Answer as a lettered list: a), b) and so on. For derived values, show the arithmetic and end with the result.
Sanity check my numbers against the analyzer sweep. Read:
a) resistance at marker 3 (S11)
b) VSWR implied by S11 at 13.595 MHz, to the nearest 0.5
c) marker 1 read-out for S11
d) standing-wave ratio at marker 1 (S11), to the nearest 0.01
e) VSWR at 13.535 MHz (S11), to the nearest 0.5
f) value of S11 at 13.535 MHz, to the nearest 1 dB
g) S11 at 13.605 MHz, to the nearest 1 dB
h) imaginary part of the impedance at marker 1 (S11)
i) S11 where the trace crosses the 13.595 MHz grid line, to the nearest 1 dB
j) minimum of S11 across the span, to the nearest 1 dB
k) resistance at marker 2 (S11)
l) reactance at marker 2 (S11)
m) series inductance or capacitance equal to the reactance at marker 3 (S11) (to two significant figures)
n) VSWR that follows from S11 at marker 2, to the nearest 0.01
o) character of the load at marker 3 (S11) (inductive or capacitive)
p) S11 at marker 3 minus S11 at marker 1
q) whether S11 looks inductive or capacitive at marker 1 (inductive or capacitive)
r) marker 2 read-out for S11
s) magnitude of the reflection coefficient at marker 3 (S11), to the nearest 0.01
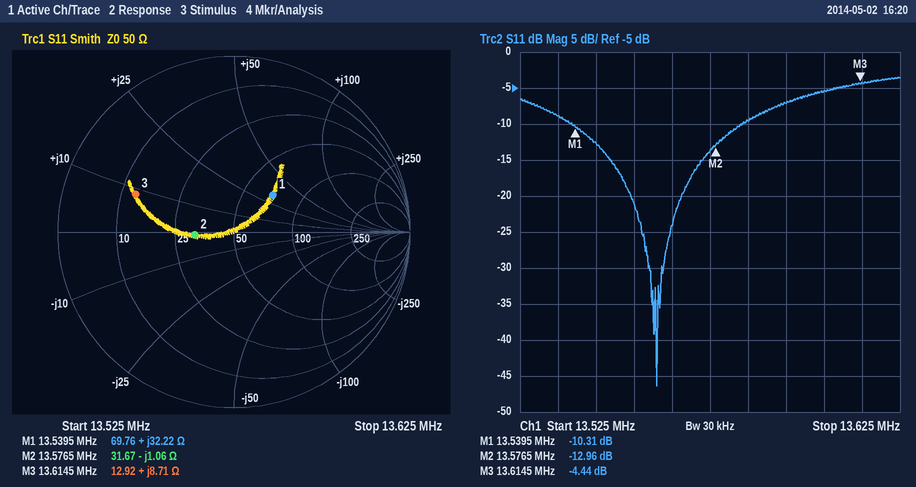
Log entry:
a) 12.92 Ω
b) |Γ| = 10^(-7/20) = 0.4467; VSWR = (1 + 0.4467)/(1 − 0.4467) ≈ 2.61, so 2.5 to the nearest 0.5
c) -10.31 dB
d) 1.88
e) |Γ| = 10^(-9/20) = 0.3548; VSWR = (1 + 0.3548)/(1 − 0.3548) ≈ 2.10, so 2.0 to the nearest 0.5
f) -9 dB
g) -5 dB
h) +32.22 Ω
i) -7 dB
j) -46 dB
k) 31.67 Ω
l) -1.06 Ω
m) L = 8.71 Ω/(2π × 13.6145 MHz) ≈ 102 nH, so 100 nH to two significant figures
n) (1 + 0.2249)/(1 − 0.2249) ≈ 1.58
o) inductive
p) -4.44 − (-10.31) = 5.87 dB
q) inductive
r) -12.96 dB
s) 10^(-4.44/20) ≈ 0.60
